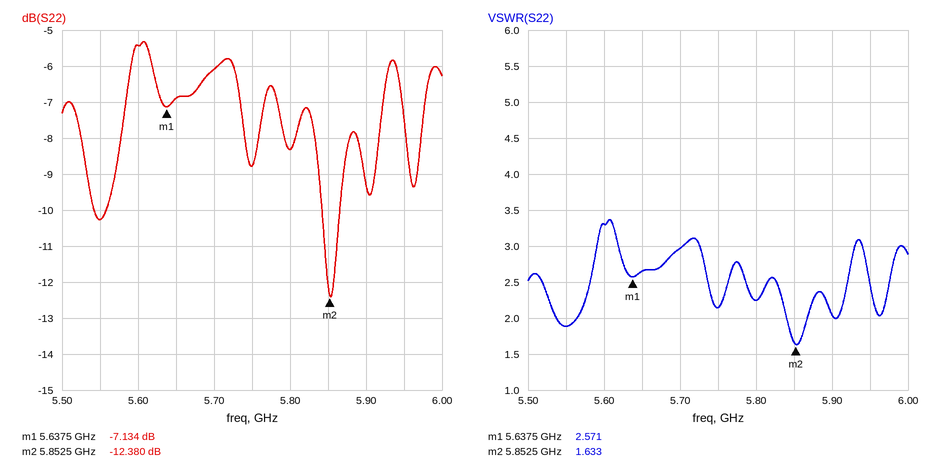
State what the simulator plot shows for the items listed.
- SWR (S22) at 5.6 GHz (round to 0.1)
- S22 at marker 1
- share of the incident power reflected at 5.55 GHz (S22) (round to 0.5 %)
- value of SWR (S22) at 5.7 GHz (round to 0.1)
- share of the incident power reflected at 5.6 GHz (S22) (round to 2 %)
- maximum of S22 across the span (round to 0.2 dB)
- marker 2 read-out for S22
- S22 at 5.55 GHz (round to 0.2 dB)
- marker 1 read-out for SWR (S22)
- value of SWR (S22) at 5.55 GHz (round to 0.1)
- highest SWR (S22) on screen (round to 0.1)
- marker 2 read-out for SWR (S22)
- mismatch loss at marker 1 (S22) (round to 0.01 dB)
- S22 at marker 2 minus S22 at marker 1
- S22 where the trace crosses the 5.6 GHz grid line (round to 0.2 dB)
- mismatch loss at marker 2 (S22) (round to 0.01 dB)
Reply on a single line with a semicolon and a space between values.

3.3; -7.134 dB; 9.5 %; 3.0; 28 %; -5.4 dB; -12.380 dB; -10.2 dB; 2.571; 1.9; 3.4; 1.633; 0.93 dB; -5.246 dB; -5.4 dB; 0.26 dB
